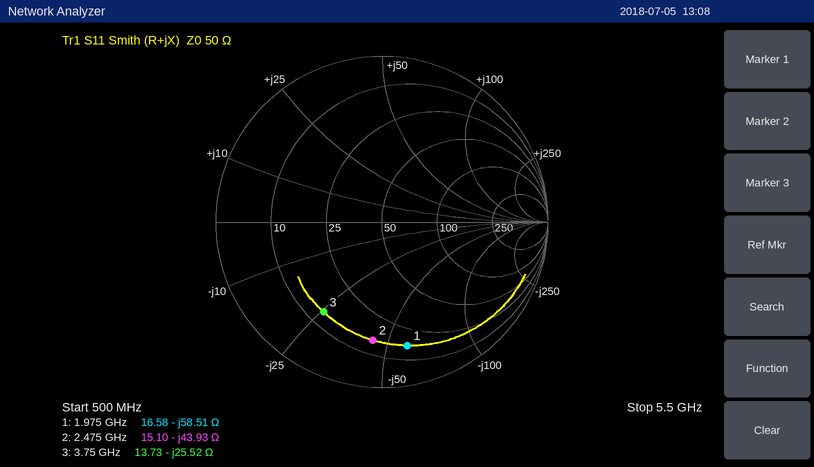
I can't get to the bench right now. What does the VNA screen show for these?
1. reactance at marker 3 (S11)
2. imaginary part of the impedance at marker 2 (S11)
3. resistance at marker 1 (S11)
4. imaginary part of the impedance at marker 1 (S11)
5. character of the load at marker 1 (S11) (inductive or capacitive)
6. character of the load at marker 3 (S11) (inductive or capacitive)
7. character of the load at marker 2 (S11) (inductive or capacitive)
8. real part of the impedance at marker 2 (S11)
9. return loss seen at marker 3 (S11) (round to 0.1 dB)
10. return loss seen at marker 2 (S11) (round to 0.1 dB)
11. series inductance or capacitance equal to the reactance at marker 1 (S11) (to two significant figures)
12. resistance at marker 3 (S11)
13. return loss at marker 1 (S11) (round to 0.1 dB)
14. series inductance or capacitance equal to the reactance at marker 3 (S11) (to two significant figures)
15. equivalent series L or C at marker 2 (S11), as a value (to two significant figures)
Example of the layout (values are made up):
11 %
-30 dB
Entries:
-25.52 Ω
-43.93 Ω
16.58 Ω
-58.51 Ω
capacitive
capacitive
capacitive
15.10 Ω
3.8 dB
2.9 dB
1.4 pF
13.73 Ω
2.4 dB
1.7 pF
1.5 pF
